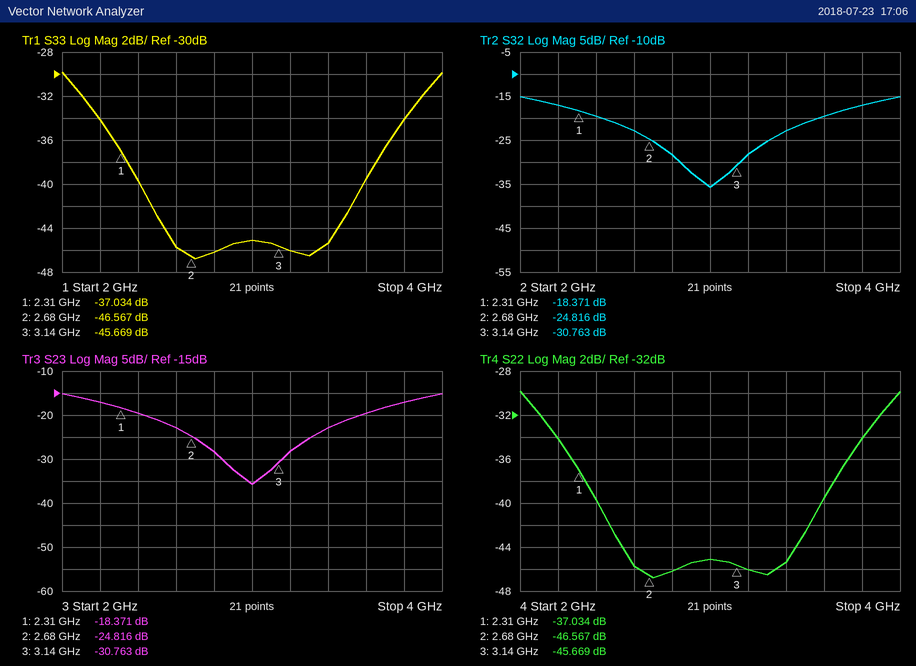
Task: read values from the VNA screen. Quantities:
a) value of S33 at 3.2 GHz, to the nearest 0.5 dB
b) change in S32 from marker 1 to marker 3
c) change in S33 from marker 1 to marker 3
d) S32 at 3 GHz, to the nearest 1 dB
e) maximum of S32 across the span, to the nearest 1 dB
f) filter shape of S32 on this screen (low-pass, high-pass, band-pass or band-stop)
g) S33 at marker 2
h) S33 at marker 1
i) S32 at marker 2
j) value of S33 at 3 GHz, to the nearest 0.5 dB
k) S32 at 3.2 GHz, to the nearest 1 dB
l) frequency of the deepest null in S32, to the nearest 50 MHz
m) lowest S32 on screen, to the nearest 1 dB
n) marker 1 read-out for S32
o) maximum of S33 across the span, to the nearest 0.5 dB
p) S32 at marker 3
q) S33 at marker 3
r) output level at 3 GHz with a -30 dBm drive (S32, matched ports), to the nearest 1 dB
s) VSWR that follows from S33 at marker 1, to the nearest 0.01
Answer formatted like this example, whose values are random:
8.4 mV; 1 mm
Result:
-46.0 dB; -12.392 dB; -8.635 dB; -36 dB; -15 dB; band-stop; -46.567 dB; -37.034 dB; -24.816 dB; -45.0 dB; -28 dB; 3.00 GHz; -36 dB; -18.371 dB; -30.0 dB; -30.763 dB; -45.669 dB; -66 dBm; 1.03
